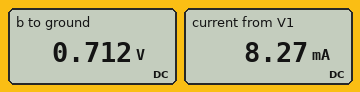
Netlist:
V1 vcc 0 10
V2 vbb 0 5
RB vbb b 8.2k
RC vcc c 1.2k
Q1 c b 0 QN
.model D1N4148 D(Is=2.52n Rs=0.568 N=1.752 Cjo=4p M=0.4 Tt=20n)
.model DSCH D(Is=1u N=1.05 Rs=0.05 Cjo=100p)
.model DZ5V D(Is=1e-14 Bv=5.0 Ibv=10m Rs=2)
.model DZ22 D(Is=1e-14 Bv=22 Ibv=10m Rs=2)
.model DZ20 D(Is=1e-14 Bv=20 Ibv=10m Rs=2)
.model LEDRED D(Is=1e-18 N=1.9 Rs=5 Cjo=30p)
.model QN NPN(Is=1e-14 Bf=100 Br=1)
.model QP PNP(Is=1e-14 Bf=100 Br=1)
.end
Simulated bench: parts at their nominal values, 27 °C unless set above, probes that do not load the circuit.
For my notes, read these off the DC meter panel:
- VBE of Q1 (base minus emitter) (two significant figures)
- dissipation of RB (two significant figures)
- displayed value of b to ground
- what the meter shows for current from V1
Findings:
710 mV
2.2 mW
0.712 V
8.27 mA
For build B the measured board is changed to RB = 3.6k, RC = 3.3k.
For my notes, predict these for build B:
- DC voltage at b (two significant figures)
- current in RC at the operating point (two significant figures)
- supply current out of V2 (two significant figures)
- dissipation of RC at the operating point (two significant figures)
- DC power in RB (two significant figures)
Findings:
700 mV
3.0 mA
1.2 mA
30 mW
5.1 mW
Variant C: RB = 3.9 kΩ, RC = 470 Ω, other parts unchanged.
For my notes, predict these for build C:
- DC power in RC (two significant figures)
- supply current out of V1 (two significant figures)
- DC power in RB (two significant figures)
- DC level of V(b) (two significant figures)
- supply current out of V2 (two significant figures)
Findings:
210 mW
21 mA
4.7 mW
740 mV
1.1 mA
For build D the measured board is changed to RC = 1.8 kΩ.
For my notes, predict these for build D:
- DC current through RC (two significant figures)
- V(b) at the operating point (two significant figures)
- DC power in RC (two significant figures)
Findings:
5.5 mA
700 mV
55 mW
